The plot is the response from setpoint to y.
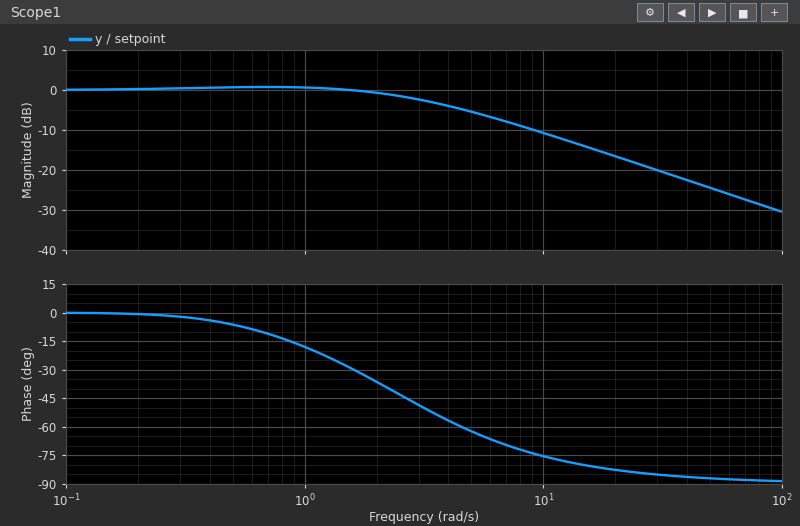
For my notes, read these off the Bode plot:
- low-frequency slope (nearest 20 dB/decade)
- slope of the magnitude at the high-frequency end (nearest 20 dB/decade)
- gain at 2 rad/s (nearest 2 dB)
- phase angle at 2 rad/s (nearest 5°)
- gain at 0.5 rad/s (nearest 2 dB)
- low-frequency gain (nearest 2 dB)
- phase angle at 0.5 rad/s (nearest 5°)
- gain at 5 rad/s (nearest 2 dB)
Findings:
0 dB/decade
-20 dB/decade
0 dB
-35°
0 dB
0 dB
-5°
-6 dB
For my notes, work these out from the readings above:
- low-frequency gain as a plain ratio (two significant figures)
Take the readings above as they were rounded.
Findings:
1.0
